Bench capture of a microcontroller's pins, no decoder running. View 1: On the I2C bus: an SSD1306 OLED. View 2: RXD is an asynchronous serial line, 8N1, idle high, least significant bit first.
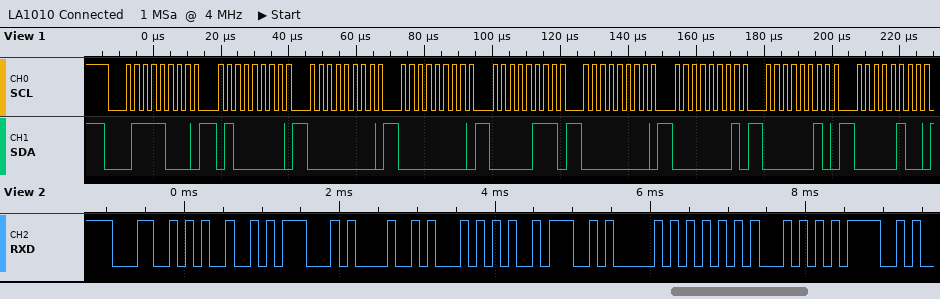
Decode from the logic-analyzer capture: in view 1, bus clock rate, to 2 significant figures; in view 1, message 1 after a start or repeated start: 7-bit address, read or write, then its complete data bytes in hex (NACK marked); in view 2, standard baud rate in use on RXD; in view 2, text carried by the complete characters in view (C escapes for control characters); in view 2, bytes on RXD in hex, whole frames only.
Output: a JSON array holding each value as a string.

["400 kHz", "0x3C write: 40 00 00 07 00 01 02 04", "9600 baud", "\"LIGHT:AUTO\"", "0x4C 0x49 0x47 0x48 0x54 0x3A 0x41 0x55 0x54 0x4F"]
